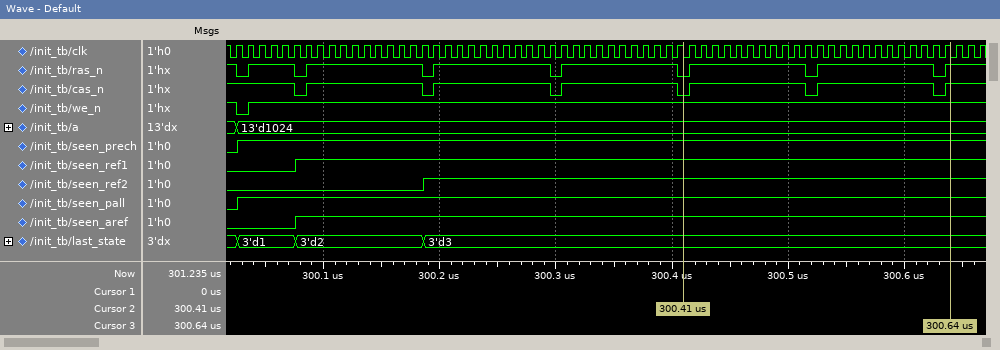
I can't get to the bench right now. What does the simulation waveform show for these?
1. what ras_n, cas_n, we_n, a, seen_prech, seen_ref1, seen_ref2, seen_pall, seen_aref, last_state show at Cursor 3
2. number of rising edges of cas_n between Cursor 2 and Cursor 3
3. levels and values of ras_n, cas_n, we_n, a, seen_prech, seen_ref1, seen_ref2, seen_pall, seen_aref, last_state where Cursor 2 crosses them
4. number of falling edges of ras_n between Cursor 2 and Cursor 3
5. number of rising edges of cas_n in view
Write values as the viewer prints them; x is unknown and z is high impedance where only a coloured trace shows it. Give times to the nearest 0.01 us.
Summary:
ras_n=1, cas_n=1, we_n=1, a=13'd1024, seen_prech=1, seen_ref1=1, seen_ref2=1, seen_pall=1, seen_aref=1, last_state=3'd3
3
ras_n=0, cas_n=0, we_n=1, a=13'd1024, seen_prech=1, seen_ref1=1, seen_ref2=1, seen_pall=1, seen_aref=1, last_state=3'd3
2
6
